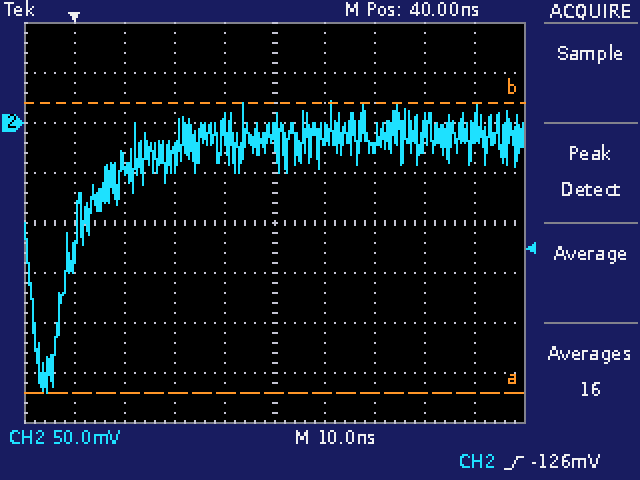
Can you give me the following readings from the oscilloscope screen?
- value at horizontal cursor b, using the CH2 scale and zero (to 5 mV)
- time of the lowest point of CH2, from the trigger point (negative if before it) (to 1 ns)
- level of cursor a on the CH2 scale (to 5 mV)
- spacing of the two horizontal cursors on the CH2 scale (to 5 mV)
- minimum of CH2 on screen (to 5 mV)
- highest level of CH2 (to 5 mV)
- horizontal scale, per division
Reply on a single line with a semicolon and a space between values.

20 mV; -6 ns; -270 mV; 290 mV; -270 mV; 20 mV; 10 ns
